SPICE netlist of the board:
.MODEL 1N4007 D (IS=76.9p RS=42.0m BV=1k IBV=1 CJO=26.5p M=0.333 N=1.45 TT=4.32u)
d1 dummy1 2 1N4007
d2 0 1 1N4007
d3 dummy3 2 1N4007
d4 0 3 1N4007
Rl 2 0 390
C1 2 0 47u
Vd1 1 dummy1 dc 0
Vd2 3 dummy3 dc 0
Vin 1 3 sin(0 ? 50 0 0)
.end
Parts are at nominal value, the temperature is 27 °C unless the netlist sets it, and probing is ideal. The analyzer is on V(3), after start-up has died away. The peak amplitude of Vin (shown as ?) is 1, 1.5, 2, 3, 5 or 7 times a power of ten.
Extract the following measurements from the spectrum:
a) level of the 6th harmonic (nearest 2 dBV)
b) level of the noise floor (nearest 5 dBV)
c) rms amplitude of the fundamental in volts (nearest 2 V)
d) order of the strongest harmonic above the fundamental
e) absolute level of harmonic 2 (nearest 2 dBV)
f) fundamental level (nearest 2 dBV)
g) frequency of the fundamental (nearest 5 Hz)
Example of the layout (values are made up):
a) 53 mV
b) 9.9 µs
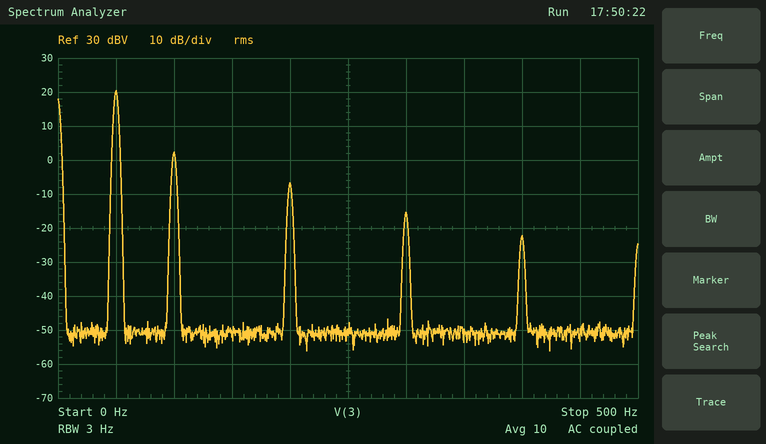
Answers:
a) -16 dBV
b) -50 dBV
c) 10 V
d) 2
e) 2 dBV
f) 20 dBV
g) 50 Hz
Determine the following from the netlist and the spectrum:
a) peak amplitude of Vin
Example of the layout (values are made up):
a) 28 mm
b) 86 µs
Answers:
a) 30 V
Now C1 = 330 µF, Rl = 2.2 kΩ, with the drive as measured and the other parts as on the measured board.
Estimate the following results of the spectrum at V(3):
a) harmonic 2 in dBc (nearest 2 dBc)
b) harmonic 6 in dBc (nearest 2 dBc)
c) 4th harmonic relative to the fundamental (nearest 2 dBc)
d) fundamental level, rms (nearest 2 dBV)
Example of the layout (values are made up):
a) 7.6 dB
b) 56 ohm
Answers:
a) -48 dBc
b) -58 dBc
c) -54 dBc
d) 20 dBV
